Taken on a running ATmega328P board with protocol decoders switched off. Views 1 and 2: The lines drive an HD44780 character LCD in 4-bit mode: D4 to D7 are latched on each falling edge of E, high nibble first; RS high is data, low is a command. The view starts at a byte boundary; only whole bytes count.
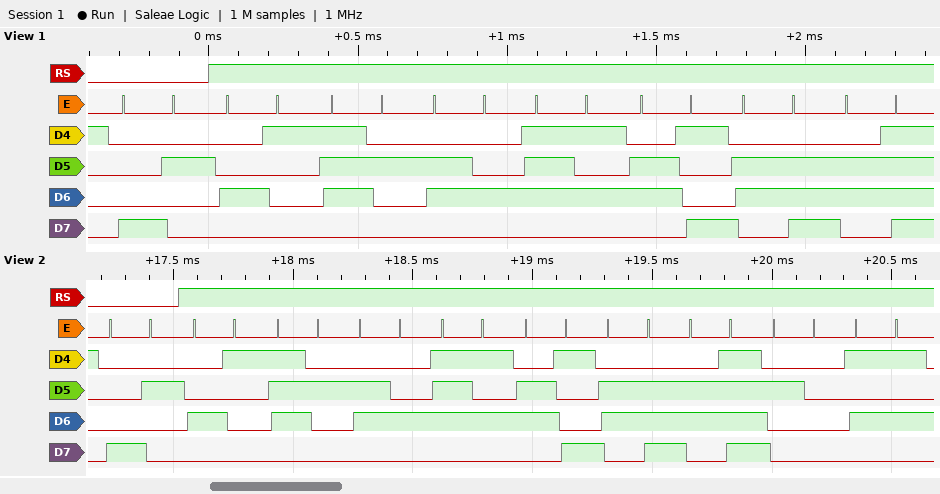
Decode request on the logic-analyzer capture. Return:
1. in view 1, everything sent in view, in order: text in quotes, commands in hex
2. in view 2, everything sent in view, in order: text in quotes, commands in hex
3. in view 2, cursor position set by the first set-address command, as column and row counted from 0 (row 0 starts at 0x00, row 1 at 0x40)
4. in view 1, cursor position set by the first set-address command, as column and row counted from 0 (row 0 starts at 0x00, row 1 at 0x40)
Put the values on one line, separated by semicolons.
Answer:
0x82 "Arduino"; 0x82 "Arduino U"; column 2, row 0; column 2, row 0
